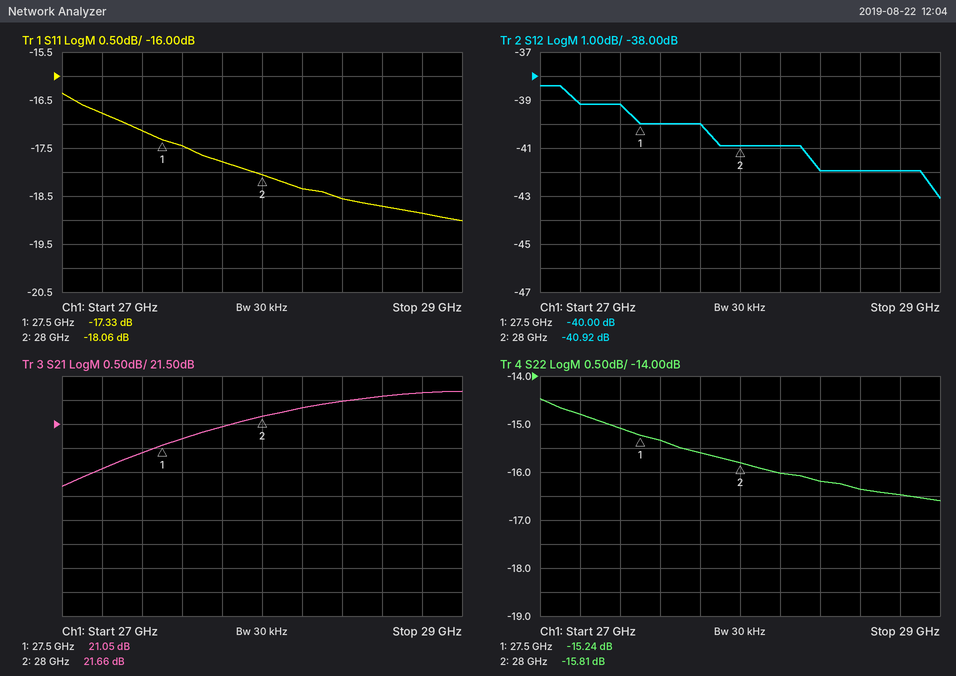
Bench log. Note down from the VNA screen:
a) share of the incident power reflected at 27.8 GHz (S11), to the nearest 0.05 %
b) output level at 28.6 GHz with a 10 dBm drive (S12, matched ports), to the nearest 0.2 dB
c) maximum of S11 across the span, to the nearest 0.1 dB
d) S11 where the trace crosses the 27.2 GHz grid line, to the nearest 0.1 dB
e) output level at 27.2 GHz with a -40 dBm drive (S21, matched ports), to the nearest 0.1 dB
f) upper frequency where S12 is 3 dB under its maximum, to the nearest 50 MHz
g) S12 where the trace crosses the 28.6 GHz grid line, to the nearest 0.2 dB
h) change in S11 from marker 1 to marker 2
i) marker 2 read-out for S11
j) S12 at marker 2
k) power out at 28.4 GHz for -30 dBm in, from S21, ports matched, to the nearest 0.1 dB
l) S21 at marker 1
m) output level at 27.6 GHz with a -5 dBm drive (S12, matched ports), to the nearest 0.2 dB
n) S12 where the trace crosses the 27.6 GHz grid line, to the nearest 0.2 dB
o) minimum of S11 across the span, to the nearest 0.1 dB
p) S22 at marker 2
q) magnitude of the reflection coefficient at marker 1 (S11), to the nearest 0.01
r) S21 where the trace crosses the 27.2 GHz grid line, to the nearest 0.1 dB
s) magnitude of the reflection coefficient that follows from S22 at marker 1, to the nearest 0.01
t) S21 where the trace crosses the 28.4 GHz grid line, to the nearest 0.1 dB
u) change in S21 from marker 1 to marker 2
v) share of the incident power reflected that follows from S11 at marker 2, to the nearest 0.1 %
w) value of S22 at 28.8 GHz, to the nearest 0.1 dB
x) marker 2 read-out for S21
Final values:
1.65 %
-32.0 dBm
-16.4 dB
-16.8 dB
-19.4 dBm
28.35 GHz
-42.0 dB
-0.73 dB
-18.06 dB
-40.92 dB
-8.0 dBm
21.05 dB
-45.0 dBm
-40.0 dB
-19.0 dB
-15.81 dB
0.14
20.6 dB
0.17
22.0 dB
0.61 dB
1.6 %
-16.5 dB
21.66 dB
